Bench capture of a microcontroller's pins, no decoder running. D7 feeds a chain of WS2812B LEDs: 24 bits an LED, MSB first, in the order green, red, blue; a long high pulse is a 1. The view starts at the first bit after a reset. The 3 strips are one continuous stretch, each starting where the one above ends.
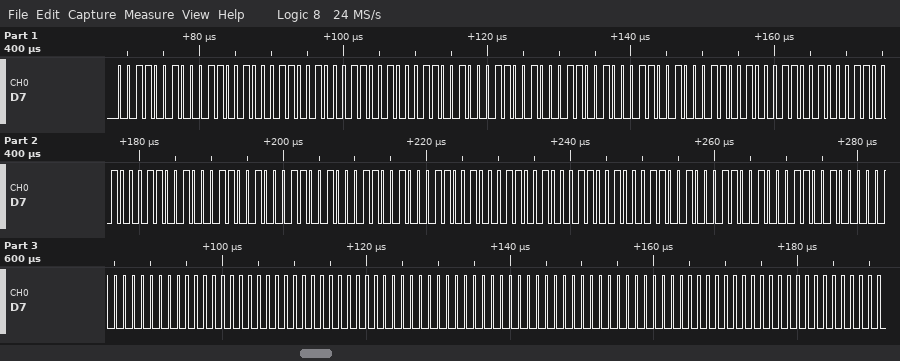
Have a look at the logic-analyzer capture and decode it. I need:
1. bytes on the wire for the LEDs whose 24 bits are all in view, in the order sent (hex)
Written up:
32 32 32 32 32 32 32 32 32 32 32 32 32 32 32 32 32 32 32 32 32 00 00 00 00 00 00 00 00 00
